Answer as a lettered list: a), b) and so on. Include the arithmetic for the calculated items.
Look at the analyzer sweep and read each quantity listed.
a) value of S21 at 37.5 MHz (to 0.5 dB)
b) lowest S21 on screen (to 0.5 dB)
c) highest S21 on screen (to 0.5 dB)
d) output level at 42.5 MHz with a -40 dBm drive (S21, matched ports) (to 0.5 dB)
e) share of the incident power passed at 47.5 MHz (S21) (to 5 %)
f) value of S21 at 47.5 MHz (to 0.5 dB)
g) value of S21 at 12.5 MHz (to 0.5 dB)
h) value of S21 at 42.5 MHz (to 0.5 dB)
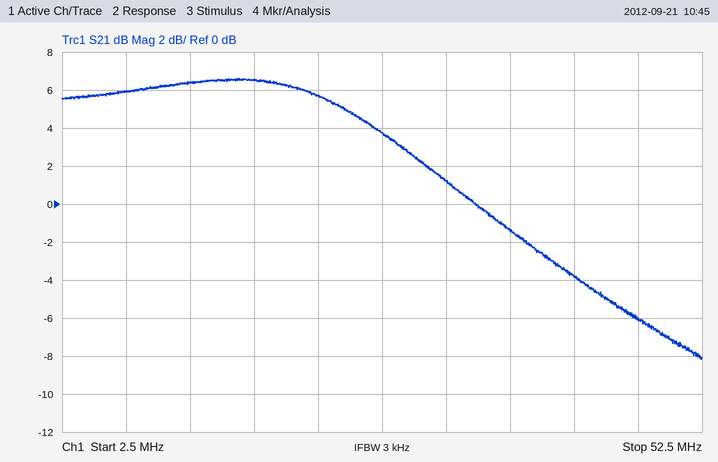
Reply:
a) -1.5 dB
b) -8.0 dB
c) 6.5 dB
d) -40 dBm + (-4.0 dB) = -44.0 dBm
e) 10^(-6/10) ≈ 25 %
f) -6.0 dB
g) 6.5 dB
h) -4.0 dB
